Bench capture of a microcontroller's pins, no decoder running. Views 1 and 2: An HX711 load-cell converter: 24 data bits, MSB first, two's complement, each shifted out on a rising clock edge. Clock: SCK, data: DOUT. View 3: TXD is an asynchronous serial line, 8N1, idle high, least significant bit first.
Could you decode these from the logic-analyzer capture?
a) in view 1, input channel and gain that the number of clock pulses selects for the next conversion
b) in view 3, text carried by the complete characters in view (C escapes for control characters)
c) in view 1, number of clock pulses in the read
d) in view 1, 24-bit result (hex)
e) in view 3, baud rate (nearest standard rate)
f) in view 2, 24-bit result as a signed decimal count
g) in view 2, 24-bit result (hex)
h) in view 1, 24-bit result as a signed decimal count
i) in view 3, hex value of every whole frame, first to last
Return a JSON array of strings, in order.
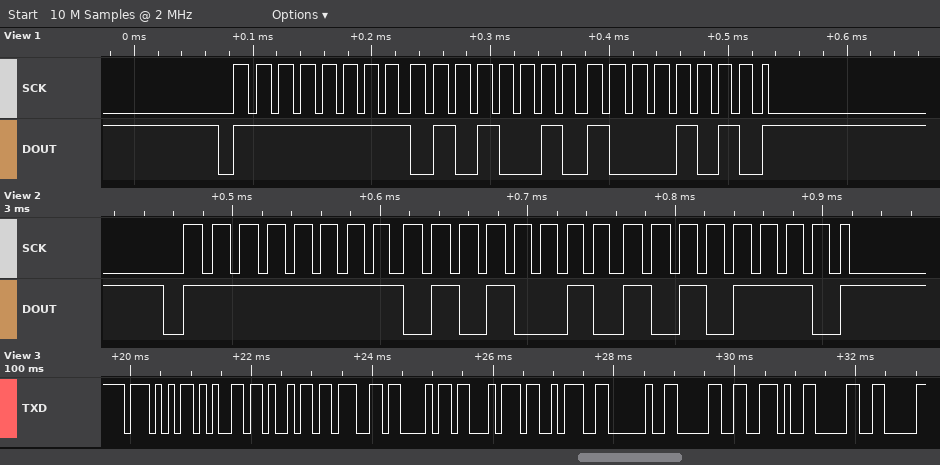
["channel A, gain 128", "\"Weight: 0.0\"", "25", "0xFF528A", "9600 baud", "-44370", "0xFF52AE", "-44406", "57 65 69 67 68 74 3A 20 30 2E 30"]
